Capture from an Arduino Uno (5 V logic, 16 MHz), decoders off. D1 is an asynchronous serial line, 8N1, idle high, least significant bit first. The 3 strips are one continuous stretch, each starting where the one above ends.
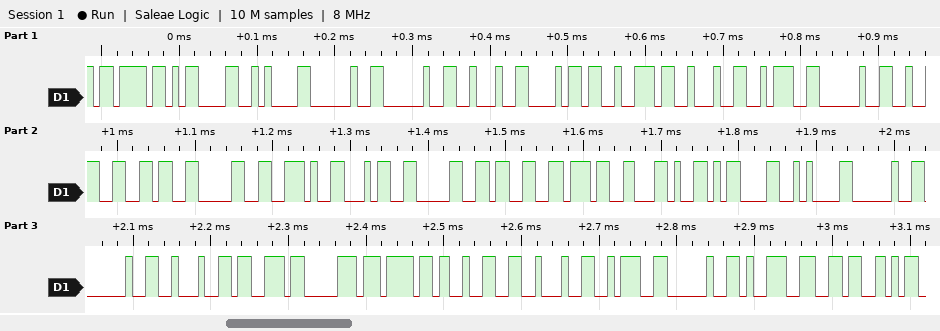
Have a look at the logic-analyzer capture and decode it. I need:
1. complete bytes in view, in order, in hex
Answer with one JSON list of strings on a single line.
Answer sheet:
["7B 0D 0A 20 20 22 68 72 22 3A 20 32 36 30 2E 34 30 33 37 2C 0D 0A 20 20 22 73 70 6F 32 22 3A 20 39 36"]
